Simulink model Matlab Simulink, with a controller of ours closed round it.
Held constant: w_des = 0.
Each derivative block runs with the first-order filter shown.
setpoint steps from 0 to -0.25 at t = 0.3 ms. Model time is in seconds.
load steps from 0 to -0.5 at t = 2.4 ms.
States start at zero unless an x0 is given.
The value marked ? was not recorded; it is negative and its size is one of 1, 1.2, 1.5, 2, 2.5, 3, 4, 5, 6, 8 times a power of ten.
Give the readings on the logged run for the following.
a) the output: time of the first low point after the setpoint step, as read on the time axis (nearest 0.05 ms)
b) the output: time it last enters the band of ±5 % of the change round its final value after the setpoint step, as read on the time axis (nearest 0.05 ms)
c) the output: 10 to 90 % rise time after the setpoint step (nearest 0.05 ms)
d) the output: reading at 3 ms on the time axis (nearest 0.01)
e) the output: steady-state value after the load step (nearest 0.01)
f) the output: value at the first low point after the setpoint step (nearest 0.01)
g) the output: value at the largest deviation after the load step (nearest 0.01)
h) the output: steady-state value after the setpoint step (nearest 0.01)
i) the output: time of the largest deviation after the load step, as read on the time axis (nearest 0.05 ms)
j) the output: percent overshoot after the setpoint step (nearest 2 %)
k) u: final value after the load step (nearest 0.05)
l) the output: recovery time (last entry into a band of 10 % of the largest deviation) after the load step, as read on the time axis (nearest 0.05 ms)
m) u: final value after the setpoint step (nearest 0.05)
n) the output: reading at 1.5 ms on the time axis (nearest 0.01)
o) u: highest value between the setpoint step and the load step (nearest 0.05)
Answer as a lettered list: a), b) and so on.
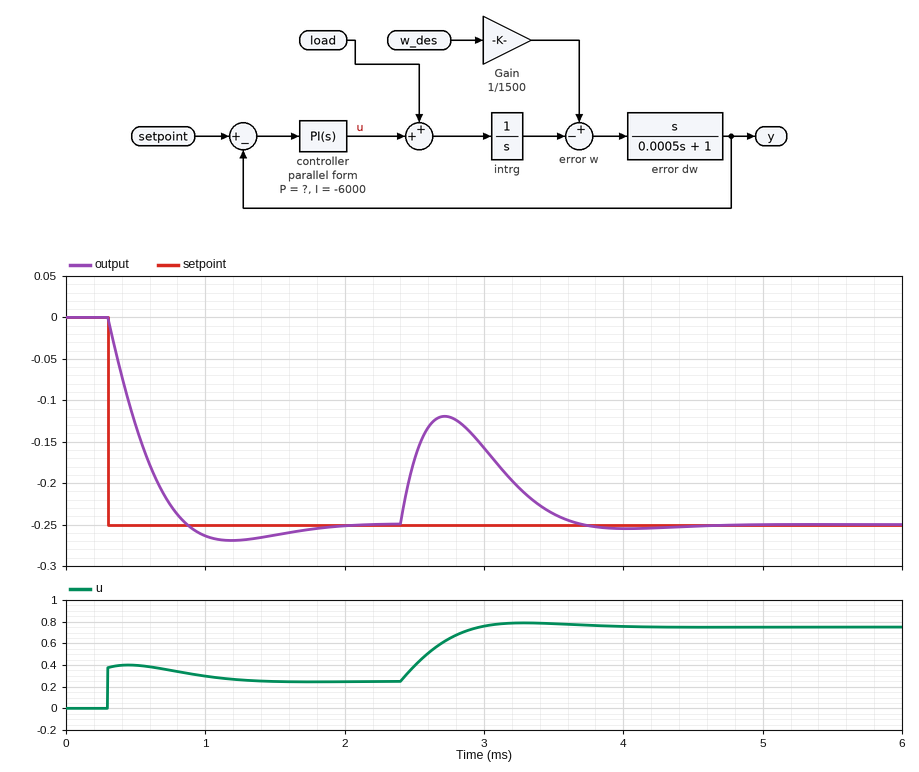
a) 1.20 ms
b) 1.50 ms
c) 0.40 ms
d) -0.16
e) -0.25
f) -0.27
g) -0.12
h) -0.25
i) 2.70 ms
j) 8 %
k) 0.75
l) 3.50 ms
m) 0.25
n) -0.26
o) 0.40
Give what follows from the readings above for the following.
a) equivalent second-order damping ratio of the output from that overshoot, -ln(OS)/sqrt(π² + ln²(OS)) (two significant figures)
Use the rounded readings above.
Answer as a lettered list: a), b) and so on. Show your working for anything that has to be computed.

a) ln(0.08) = -2.526; 2.526 / sqrt(9.870 + 6.379) = 0.63
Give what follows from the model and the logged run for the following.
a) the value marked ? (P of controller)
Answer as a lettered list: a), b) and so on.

a) -1.5
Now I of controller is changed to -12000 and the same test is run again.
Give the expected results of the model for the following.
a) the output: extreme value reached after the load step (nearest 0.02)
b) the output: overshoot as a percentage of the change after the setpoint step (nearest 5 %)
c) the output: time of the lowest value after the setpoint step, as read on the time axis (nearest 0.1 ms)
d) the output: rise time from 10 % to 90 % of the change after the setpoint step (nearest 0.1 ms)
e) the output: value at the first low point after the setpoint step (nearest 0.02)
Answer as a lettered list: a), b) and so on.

a) -0.14
b) 20 %
c) 0.9 ms
d) 0.3 ms
e) -0.30
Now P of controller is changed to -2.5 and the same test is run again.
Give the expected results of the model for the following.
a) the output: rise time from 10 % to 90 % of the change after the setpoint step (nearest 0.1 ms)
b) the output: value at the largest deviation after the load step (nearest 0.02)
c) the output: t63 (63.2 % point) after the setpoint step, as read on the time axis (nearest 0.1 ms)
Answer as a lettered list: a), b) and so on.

a) 0.4 ms
b) -0.14
c) 0.5 ms
